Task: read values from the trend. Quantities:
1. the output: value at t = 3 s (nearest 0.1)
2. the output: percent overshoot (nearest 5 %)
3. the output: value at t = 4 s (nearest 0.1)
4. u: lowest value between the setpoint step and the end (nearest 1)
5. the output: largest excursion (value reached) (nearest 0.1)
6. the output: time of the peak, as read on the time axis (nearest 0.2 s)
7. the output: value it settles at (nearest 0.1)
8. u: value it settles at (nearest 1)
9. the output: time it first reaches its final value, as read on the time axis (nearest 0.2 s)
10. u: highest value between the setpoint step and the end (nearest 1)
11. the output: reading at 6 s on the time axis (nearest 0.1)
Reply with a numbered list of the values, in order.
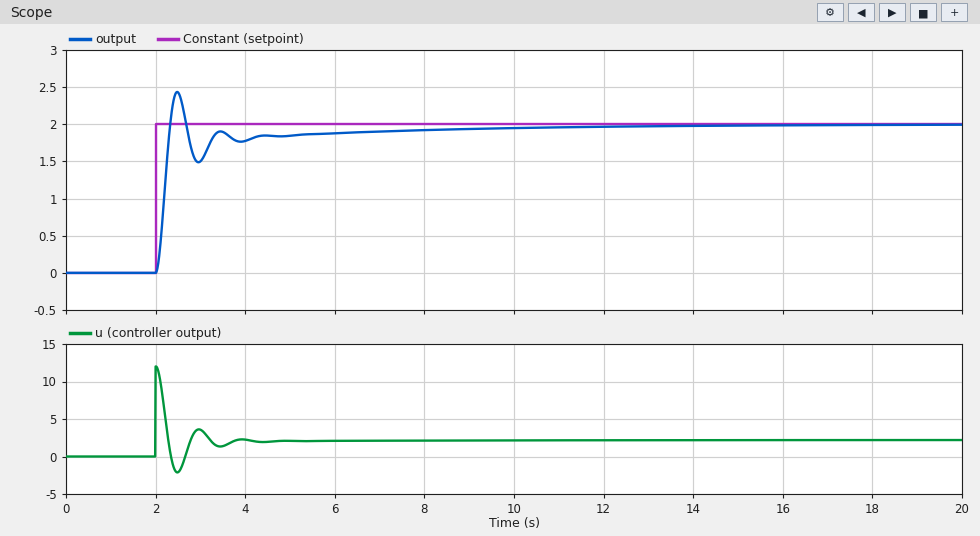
1. 1.5
2. 20 %
3. 1.8
4. -2
5. 2.4
6. 2.4 s
7. 2.0
8. 2
9. 2.4 s
10. 12
11. 1.9
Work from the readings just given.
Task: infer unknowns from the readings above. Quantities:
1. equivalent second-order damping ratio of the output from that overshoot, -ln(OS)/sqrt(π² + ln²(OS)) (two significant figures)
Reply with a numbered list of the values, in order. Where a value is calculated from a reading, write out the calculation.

1. ln(0.2) = -1.609; 1.609 / sqrt(9.870 + 2.590) = 0.46
